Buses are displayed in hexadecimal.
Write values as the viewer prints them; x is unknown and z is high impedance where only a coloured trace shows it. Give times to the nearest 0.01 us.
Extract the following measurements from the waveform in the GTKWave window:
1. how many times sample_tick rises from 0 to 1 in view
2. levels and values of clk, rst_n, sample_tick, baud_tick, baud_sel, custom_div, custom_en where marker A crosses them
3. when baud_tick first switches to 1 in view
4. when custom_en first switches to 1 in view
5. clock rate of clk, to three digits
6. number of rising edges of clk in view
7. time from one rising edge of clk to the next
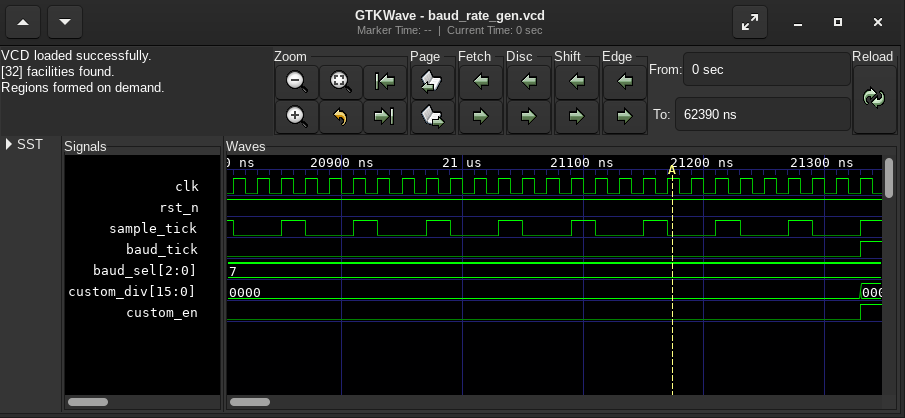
9
clk=1, rst_n=1, sample_tick=0, baud_tick=0, baud_sel=7, custom_div=0000, custom_en=0
21.33 us
21.33 us
50.0 MHz
27
0.02 us
